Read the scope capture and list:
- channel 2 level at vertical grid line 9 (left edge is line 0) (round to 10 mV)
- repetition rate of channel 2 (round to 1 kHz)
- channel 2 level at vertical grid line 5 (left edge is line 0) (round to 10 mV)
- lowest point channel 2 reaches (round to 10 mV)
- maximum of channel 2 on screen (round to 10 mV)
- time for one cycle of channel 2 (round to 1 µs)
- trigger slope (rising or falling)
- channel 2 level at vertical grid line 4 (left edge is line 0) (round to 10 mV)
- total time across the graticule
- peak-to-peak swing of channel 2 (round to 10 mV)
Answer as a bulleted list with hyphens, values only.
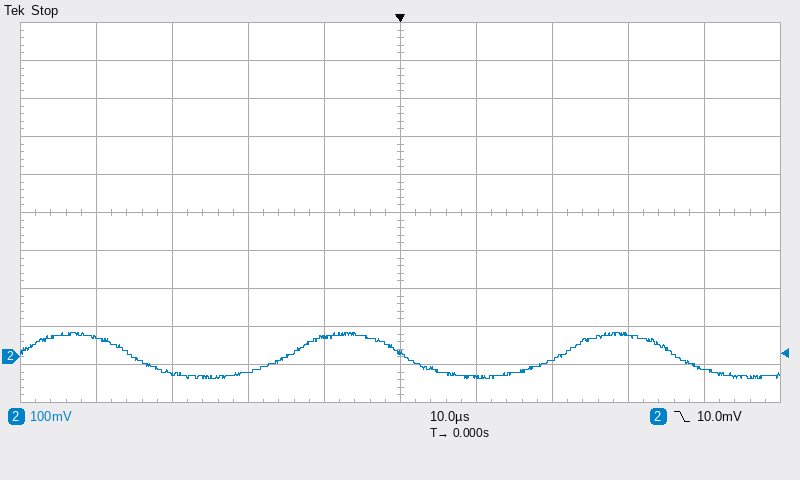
- -30 mV
- 28 kHz
- 10 mV
- -60 mV
- 60 mV
- 36 µs
- falling
- 50 mV
- 100 µs
- 120 mV
